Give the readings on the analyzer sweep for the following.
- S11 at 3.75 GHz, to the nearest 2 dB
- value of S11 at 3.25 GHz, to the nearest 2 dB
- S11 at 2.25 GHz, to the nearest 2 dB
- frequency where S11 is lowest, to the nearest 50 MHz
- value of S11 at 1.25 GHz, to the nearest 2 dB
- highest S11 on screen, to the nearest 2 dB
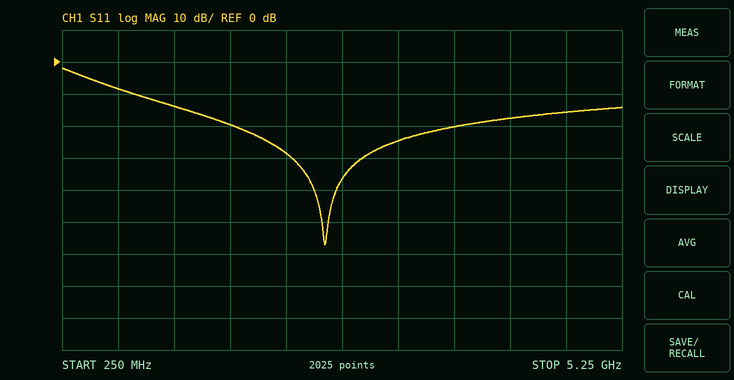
-20 dB
-24 dB
-28 dB
2.60 GHz
-14 dB
-2 dB
